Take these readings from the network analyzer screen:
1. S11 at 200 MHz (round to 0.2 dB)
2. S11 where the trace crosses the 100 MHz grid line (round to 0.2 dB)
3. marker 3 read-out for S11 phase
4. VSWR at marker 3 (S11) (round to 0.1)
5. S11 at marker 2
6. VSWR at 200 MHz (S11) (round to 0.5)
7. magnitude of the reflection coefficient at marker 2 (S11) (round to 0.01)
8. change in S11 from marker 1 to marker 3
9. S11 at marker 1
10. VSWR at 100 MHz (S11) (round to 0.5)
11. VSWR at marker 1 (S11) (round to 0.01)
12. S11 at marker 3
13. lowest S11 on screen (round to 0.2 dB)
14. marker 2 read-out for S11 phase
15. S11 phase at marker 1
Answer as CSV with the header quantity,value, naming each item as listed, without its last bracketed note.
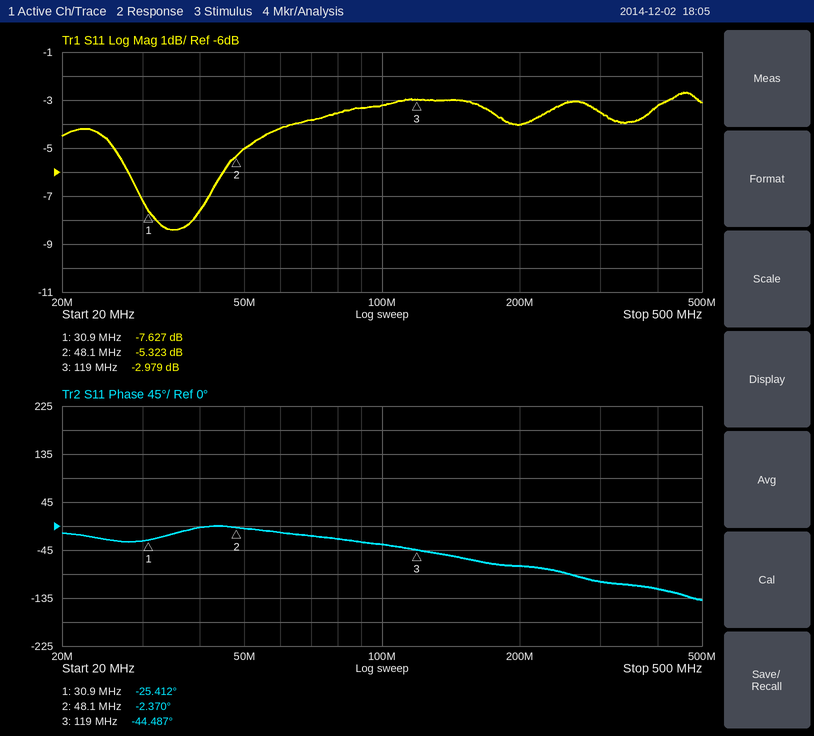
quantity,value
S11 at 200 MHz,-4.0 dB
S11 where the trace crosses the 100 MHz grid line,-3.2 dB
marker 3 read-out for S11 phase,-44.487°
VSWR at marker 3 (S11),5.9
S11 at marker 2,-5.323 dB
VSWR at 200 MHz (S11),4.5
magnitude of the reflection coefficient at marker 2 (S11),0.54
change in S11 from marker 1 to marker 3,4.648 dB
S11 at marker 1,-7.627 dB
VSWR at 100 MHz (S11),5.5
VSWR at marker 1 (S11),2.42
S11 at marker 3,-2.979 dB
lowest S11 on screen,-8.4 dB
marker 2 read-out for S11 phase,-2.370°
S11 phase at marker 1,-25.412°
